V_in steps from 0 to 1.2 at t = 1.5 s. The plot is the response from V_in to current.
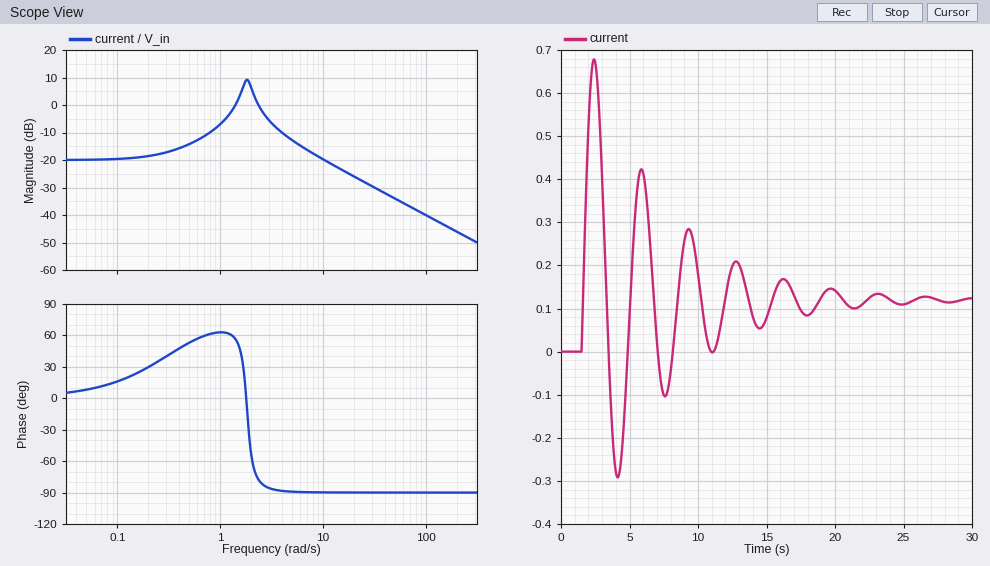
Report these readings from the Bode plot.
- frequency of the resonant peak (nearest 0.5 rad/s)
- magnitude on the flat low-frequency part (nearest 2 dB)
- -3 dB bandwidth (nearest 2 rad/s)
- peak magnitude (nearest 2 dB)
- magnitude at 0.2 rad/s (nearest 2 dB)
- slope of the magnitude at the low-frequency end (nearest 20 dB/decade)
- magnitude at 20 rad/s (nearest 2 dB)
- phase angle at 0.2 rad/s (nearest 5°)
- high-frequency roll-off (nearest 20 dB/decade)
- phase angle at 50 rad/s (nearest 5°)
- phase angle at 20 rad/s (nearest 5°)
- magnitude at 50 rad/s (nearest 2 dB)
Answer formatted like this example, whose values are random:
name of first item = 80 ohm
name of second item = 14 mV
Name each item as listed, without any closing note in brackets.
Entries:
frequency of the resonant peak = 2.0 rad/s
magnitude on the flat low-frequency part = -20 dB
-3 dB bandwidth = 14 rad/s
peak magnitude = 10 dB
magnitude at 0.2 rad/s = -18 dB
slope of the magnitude at the low-frequency end = 0 dB/decade
magnitude at 20 rad/s = -26 dB
phase angle at 0.2 rad/s = 30°
high-frequency roll-off = -20 dB/decade
phase angle at 50 rad/s = -90°
phase angle at 20 rad/s = -90°
magnitude at 50 rad/s = -34 dB
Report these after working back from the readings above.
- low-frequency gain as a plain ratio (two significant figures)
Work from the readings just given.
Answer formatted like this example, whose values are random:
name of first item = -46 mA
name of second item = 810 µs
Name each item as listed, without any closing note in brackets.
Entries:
low-frequency gain as a plain ratio = 0.10
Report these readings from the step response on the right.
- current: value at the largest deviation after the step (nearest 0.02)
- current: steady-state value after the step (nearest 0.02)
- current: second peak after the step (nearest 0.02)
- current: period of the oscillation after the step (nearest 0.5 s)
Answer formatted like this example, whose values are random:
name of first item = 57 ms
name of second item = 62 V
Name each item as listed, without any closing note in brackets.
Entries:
current: value at the largest deviation after the step = 0.68
current: steady-state value after the step = 0.12
current: second peak after the step = 0.42
current: period of the oscillation after the step = 3.5 s
